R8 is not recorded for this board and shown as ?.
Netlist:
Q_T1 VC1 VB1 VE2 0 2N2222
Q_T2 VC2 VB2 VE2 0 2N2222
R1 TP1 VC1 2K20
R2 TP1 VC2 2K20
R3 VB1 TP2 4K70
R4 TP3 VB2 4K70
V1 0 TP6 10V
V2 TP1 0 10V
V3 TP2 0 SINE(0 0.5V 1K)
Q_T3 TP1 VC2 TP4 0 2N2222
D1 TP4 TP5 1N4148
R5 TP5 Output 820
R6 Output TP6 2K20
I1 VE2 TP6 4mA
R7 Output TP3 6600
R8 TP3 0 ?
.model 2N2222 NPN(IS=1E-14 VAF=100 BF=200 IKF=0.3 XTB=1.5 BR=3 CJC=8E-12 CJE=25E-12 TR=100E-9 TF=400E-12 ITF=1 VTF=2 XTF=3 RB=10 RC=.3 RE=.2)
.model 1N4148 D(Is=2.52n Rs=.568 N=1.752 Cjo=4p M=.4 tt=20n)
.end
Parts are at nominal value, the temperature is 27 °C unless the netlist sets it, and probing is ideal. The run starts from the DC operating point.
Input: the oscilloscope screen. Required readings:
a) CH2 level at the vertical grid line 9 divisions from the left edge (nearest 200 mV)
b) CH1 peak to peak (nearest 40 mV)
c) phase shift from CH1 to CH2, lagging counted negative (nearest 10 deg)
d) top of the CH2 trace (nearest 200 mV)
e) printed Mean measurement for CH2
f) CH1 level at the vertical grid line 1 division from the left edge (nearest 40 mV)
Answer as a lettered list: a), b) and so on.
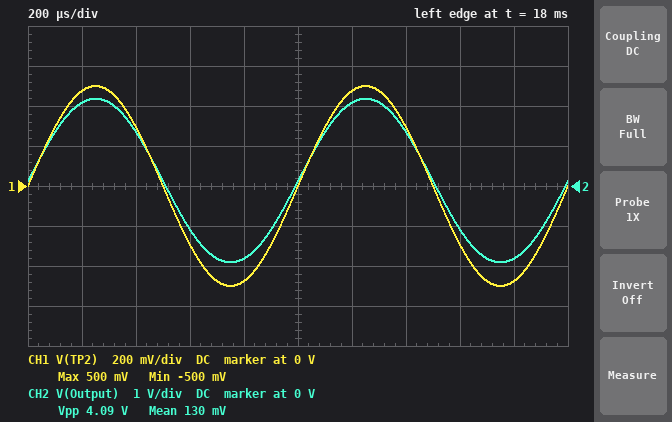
a) -1.8 V
b) 1.00 V
c) 0 deg
d) 2.2 V
e) 130 mV
f) 480 mV
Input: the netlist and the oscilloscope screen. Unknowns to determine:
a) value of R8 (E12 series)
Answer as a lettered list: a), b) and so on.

a) 1.5 kΩ
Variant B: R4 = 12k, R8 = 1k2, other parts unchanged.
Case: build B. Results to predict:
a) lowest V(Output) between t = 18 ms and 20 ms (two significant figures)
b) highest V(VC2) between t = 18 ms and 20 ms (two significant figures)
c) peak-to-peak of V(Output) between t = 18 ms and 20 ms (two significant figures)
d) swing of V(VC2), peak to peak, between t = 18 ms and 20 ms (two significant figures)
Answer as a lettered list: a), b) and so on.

a) -1.7 V
b) 8.9 V
c) 4.2 V
d) 6.3 V
